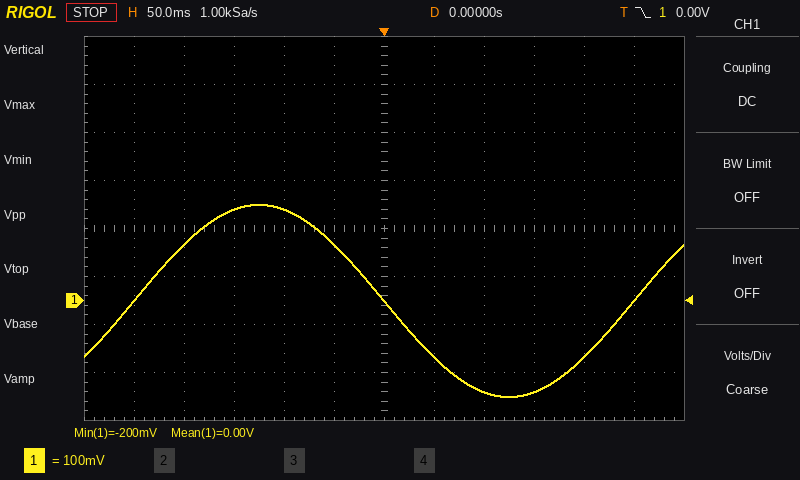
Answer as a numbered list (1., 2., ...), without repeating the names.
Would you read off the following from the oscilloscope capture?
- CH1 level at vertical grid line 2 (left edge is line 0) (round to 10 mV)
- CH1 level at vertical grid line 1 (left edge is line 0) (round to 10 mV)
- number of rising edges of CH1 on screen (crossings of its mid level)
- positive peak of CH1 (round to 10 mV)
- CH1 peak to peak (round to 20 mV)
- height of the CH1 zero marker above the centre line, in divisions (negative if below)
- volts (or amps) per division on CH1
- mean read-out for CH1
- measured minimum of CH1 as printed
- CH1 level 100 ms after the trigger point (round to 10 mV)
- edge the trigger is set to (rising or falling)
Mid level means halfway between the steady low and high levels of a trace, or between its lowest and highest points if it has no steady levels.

1. 120 mV
2. 0 mV
3. 2
4. 200 mV
5. 400 mV
6. -1.5 div
7. 100 mV
8. 0.00 V
9. -200 mV
10. -190 mV
11. falling
